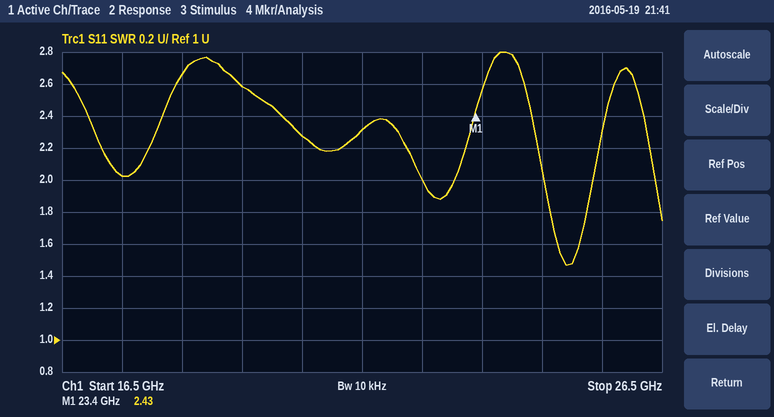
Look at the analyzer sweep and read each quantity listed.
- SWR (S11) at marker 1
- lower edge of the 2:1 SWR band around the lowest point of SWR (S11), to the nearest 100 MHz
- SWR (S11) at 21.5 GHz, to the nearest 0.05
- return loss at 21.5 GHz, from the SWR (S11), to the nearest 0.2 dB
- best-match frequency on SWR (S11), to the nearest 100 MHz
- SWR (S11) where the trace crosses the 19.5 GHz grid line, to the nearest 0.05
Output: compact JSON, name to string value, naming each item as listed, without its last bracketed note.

{"SWR (S11) at marker 1": "2.43", "lower edge of the 2:1 SWR band around the lowest point of SWR (S11), to the nearest 100 MHz": "24.5 GHz", "SWR (S11) at 21.5 GHz, to the nearest 0.05": "2.30", "return loss at 21.5 GHz, from the SWR (S11), to the nearest 0.2 dB": "8.0 dB", "best-match frequency on SWR (S11), to the nearest 100 MHz": "24.9 GHz", "SWR (S11) where the trace crosses the 19.5 GHz grid line, to the nearest 0.05": "2.60"}
